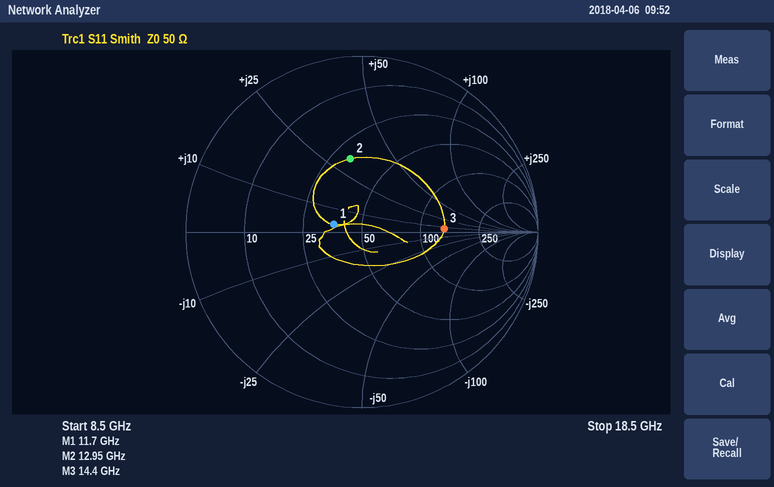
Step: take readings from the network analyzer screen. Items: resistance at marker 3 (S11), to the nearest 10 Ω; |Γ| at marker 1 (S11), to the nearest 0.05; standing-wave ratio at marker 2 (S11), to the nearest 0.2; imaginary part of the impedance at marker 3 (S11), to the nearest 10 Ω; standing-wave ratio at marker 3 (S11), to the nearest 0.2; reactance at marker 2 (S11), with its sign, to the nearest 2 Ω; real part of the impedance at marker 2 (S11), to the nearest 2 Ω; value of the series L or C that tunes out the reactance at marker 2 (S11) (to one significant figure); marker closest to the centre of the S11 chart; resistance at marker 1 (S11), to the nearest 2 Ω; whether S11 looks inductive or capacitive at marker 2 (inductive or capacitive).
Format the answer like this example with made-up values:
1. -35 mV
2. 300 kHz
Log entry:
1. 140 Ω
2. 0.15
3. 2.4
4. +10 Ω
5. 2.8
6. +32 Ω
7. 32 Ω
8. 400 fF
9. marker 1
10. 36 Ω
11. inductive
